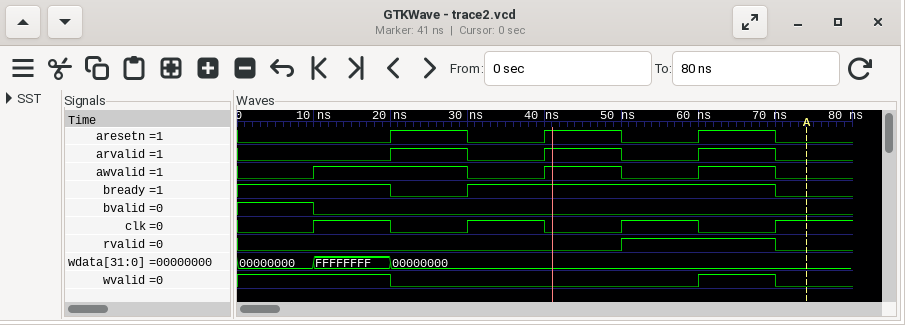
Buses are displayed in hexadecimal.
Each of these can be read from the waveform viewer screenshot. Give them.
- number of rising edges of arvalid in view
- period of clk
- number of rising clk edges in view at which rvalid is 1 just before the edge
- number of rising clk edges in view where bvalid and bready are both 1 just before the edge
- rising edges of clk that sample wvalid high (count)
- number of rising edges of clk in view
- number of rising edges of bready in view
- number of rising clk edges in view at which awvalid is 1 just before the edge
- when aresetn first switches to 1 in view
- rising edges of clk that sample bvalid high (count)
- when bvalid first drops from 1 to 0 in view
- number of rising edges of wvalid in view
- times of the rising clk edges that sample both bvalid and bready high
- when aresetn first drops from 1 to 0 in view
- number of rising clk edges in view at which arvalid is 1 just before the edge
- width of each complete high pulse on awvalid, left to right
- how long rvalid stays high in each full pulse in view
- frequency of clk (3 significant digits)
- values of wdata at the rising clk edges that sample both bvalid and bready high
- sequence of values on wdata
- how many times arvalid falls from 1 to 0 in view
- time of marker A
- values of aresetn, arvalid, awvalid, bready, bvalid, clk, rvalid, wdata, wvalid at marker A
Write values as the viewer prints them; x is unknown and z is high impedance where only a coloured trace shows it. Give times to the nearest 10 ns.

3
20 ns
1
1
2
4
1
3
20 ns
1
10 ns
1
10 ns
30 ns
3
20 ns, 10 ns, 10 ns
20 ns
50.0 MHz
00000000
00000000, FFFFFFFF, 00000000
3
70 ns
aresetn=0, arvalid=0, awvalid=0, bready=0, bvalid=0, clk=1, rvalid=0, wdata=00000000, wvalid=0
